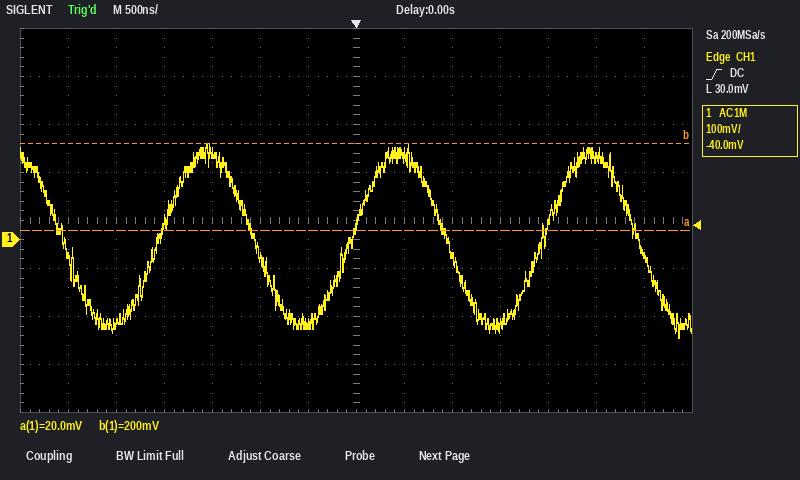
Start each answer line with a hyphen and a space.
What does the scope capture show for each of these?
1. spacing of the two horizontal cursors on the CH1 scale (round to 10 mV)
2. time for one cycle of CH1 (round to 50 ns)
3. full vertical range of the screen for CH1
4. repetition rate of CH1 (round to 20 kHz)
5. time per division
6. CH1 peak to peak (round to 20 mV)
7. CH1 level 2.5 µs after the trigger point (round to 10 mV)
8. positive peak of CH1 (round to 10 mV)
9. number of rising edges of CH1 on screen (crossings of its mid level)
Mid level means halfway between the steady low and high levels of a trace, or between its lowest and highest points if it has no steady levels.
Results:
- 180 mV
- 2.00 µs
- 800 mV
- 500 kHz
- 500 ns
- 400 mV
- 170 mV
- 200 mV
- 3
